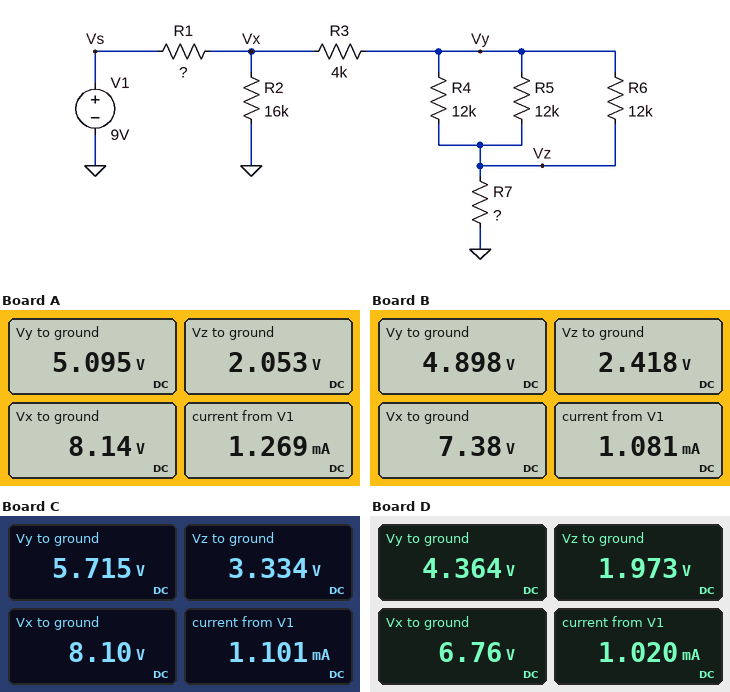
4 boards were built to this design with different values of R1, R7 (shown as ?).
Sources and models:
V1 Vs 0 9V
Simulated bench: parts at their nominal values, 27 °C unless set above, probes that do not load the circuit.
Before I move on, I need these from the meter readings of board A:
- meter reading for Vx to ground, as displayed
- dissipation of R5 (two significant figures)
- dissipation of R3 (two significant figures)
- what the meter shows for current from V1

8.14 V
770 µW
2.3 mW
1.269 mA
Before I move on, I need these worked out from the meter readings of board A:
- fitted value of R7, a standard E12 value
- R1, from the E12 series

2.7 kΩ
680 Ω
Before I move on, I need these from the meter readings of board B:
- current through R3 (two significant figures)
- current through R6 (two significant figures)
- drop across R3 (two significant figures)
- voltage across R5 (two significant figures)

620 µA
210 µA
2.5 V
2.5 V
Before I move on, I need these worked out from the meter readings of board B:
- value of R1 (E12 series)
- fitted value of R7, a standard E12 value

1.5 kΩ
3.9 kΩ
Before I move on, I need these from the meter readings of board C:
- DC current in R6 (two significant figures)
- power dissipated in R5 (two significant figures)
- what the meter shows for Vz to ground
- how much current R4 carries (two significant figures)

200 µA
470 µW
3.334 V
200 µA
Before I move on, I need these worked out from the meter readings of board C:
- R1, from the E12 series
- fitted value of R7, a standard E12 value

820 Ω
5.6 kΩ
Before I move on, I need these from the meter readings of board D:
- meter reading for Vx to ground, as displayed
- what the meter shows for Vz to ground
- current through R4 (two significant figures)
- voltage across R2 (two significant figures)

6.76 V
1.973 V
200 µA
6.8 V
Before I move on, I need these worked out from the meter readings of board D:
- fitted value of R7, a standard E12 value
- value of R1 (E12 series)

3.3 kΩ
2.2 kΩ
